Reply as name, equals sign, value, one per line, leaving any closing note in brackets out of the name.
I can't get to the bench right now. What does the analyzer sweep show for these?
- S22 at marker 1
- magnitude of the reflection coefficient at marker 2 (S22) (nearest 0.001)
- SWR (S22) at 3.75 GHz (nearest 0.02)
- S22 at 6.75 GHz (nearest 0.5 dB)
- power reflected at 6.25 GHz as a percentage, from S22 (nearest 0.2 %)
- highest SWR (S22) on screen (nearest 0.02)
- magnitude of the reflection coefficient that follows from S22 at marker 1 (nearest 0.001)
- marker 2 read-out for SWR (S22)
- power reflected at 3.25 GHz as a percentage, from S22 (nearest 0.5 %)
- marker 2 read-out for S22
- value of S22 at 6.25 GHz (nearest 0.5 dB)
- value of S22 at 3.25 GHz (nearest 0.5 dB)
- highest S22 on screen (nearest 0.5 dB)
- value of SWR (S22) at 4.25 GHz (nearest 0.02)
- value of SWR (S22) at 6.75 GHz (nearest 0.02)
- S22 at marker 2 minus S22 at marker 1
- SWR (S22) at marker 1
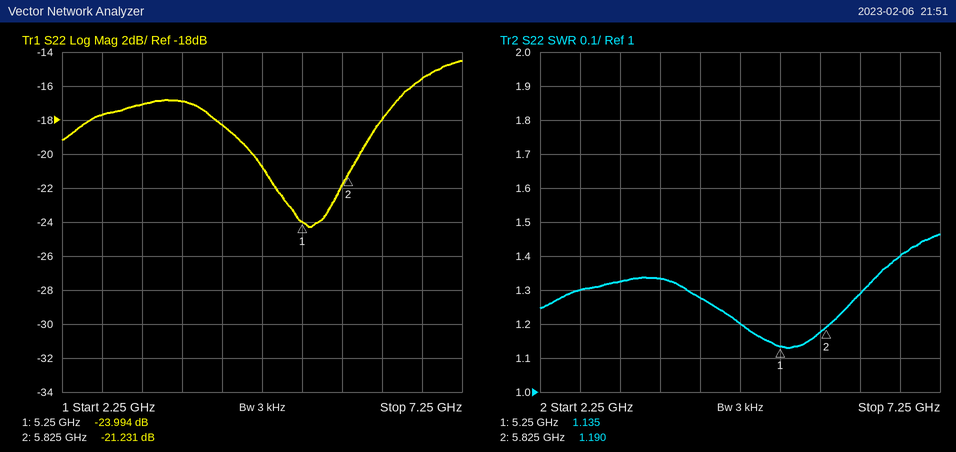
S22 at marker 1 = -23.994 dB
magnitude of the reflection coefficient at marker 2 (S22) = 0.087
SWR (S22) at 3.75 GHz = 1.34
S22 at 6.75 GHz = -15.5 dB
power reflected at 6.25 GHz as a percentage, from S22 = 1.6 %
highest SWR (S22) on screen = 1.46
magnitude of the reflection coefficient that follows from S22 at marker 1 = 0.063
marker 2 read-out for SWR = 1.190
power reflected at 3.25 GHz as a percentage, from S22 = 2.0 %
marker 2 read-out for S22 = -21.231 dB
value of S22 at 6.25 GHz = -18.0 dB
value of S22 at 3.25 GHz = -17.0 dB
highest S22 on screen = -14.5 dB
value of SWR (S22) at 4.25 GHz = 1.28
value of SWR (S22) at 6.75 GHz = 1.40
S22 at marker 2 minus S22 at marker 1 = 2.763 dB
SWR (S22) at marker 1 = 1.135
